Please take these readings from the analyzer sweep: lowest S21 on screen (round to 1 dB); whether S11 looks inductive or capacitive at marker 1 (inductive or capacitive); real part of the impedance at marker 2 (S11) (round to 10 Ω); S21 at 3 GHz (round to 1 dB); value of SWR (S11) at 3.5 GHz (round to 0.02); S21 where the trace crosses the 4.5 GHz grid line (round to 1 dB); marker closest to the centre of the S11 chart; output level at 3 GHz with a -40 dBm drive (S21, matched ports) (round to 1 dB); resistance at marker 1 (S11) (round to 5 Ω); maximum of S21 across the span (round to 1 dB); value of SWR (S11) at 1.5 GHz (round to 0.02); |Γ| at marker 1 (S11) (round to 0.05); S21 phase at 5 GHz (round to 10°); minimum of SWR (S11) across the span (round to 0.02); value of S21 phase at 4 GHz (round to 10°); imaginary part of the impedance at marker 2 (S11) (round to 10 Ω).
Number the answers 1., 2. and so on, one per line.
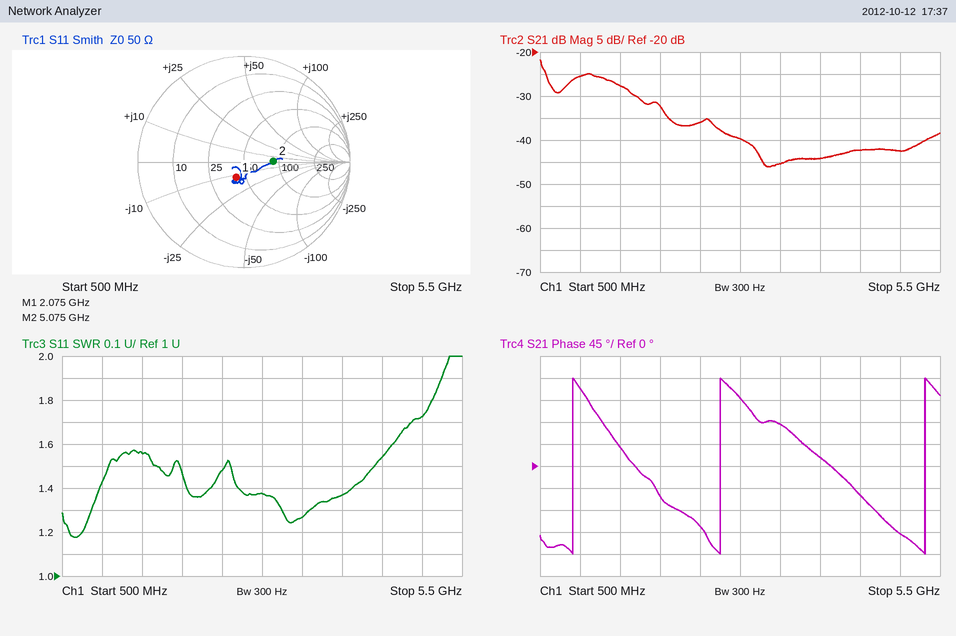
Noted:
1. -46 dB
2. capacitive
3. 90 Ω
4. -40 dB
5. 1.26
6. -42 dB
7. marker 1
8. -80 dBm
9. 40 Ω
10. -22 dB
11. 1.56
12. 0.15
13. -140°
14. 1.18
15. 20°
16. 0 Ω
